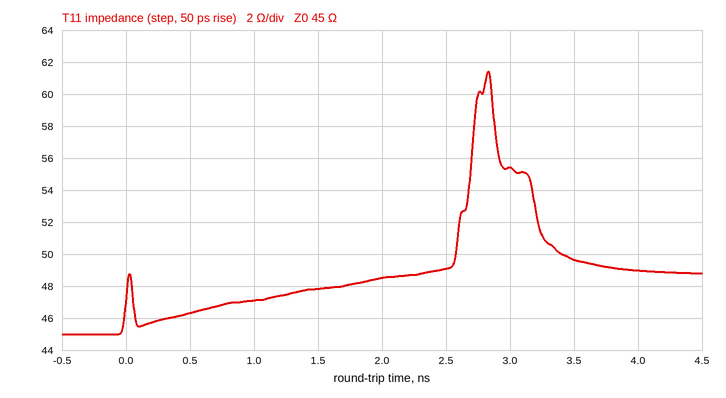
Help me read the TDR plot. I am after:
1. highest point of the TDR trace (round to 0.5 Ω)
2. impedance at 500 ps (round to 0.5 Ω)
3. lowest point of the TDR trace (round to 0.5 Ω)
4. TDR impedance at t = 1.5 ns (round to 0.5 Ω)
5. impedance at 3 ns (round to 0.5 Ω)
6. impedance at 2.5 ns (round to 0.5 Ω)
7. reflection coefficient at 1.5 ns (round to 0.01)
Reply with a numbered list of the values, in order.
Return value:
1. 61.5 Ω
2. 46.5 Ω
3. 45.0 Ω
4. 48.0 Ω
5. 55.5 Ω
6. 49.0 Ω
7. +0.03
